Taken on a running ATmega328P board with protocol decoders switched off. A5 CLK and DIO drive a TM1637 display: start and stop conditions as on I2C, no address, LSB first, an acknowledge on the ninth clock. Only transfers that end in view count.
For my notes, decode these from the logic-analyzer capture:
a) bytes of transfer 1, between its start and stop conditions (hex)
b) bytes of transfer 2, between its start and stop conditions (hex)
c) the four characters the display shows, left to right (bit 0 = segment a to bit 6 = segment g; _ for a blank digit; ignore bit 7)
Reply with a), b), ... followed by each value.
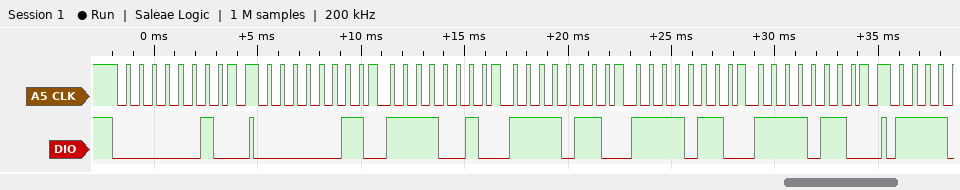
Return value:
a) 40
b) C0 4F 6F 6F 6F
c) 3999
